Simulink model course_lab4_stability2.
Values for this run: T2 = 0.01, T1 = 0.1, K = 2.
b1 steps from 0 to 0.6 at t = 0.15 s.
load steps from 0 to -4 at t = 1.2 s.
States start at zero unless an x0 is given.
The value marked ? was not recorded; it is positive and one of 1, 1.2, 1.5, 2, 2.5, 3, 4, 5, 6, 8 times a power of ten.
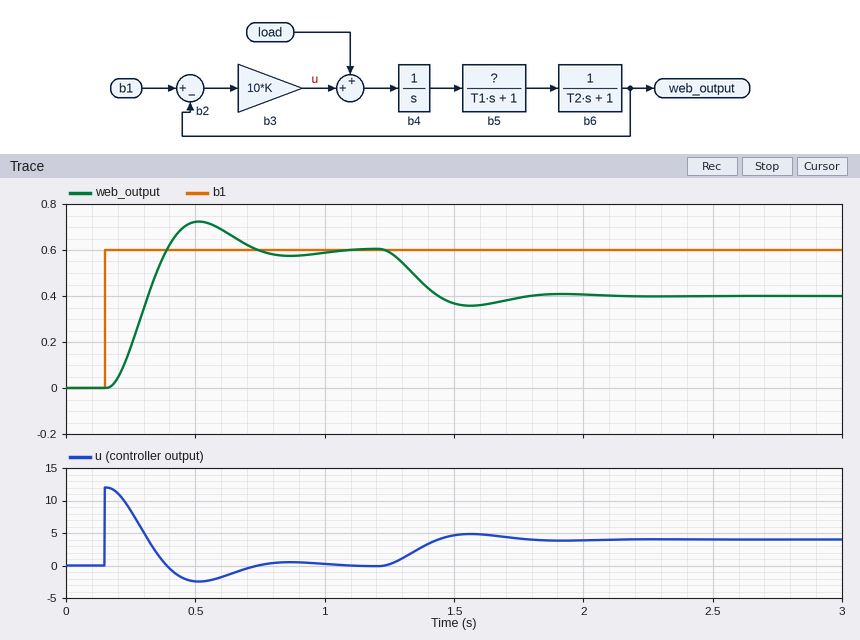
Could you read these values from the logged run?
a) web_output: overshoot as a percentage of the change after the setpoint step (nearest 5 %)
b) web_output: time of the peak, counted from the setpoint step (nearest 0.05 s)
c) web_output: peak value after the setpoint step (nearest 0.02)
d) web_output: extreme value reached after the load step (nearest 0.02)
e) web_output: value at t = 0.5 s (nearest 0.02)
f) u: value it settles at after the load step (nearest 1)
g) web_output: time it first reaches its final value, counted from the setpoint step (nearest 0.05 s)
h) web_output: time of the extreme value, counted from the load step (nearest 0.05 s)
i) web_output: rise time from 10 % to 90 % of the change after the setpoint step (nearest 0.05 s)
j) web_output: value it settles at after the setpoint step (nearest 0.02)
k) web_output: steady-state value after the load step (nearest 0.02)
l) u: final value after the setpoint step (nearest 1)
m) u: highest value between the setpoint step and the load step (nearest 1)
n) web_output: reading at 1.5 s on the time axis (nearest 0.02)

20 %
0.35 s
0.72
0.36
0.72
4
0.25 s
0.35 s
0.15 s
0.60
0.40
0
12
0.36
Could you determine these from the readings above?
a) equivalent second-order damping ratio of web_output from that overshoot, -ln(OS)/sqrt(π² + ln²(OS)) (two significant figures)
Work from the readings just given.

0.46
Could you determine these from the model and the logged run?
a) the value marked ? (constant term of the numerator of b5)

0.5
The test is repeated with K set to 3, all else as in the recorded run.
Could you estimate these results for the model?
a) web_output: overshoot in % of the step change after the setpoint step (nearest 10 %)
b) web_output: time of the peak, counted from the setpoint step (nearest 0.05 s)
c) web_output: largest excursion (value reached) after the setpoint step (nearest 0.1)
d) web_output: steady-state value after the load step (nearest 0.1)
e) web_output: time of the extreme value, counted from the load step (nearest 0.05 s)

30 %
0.30 s
0.8
0.5
0.30 s
